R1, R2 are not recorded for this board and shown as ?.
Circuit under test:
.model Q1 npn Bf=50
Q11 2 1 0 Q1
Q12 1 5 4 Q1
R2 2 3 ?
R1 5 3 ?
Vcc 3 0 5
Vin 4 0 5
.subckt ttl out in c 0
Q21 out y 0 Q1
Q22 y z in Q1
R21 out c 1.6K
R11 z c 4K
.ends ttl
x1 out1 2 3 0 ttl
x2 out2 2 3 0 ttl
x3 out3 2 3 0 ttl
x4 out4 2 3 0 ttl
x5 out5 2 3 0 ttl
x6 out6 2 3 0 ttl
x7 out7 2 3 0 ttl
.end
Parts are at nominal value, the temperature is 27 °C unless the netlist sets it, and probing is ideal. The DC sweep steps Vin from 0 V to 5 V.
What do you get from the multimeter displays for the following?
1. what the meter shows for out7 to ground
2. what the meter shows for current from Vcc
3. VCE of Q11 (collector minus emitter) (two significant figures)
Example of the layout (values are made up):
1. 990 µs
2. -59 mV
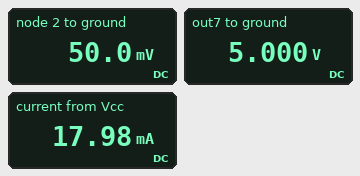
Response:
1. 5.000 V
2. 17.98 mA
3. 50 mV
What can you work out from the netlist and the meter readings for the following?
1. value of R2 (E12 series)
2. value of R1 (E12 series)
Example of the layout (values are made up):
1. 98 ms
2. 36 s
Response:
1. 560 Ω
2. 1.8 kΩ
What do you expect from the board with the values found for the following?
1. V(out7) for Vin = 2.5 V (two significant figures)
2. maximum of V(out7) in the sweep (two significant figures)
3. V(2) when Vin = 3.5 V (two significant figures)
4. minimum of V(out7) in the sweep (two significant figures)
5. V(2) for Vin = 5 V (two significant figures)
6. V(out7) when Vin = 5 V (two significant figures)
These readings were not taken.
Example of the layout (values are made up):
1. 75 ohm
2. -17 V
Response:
1. 5.0 V
2. 5.0 V
3. 50 mV
4. 36 mV
5. 50 mV
6. 5.0 V
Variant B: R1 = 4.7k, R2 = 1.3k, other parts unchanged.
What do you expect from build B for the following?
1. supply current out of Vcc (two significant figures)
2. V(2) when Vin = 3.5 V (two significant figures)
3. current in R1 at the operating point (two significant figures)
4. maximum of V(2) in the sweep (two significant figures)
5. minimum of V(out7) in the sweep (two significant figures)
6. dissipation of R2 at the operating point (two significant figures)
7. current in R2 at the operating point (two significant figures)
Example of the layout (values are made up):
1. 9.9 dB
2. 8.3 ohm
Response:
1. 12 mA
2. 63 mV
3. 720 µA
4. 840 mV
5. 39 mV
6. 19 mW
7. 3.8 mA
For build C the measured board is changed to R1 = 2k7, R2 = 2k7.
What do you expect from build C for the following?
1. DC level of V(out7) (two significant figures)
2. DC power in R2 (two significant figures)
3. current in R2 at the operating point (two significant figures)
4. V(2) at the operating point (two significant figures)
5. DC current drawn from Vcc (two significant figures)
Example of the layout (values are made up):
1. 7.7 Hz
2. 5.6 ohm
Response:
1. 5.0 V
2. 9.1 mW
3. 1.8 mA
4. 47 mV
5. 10 mA
